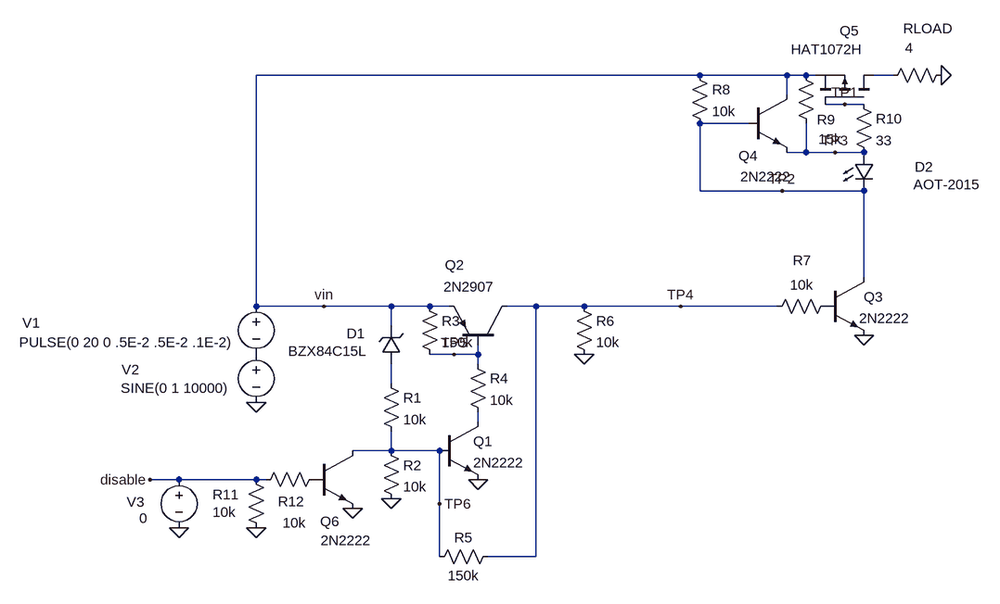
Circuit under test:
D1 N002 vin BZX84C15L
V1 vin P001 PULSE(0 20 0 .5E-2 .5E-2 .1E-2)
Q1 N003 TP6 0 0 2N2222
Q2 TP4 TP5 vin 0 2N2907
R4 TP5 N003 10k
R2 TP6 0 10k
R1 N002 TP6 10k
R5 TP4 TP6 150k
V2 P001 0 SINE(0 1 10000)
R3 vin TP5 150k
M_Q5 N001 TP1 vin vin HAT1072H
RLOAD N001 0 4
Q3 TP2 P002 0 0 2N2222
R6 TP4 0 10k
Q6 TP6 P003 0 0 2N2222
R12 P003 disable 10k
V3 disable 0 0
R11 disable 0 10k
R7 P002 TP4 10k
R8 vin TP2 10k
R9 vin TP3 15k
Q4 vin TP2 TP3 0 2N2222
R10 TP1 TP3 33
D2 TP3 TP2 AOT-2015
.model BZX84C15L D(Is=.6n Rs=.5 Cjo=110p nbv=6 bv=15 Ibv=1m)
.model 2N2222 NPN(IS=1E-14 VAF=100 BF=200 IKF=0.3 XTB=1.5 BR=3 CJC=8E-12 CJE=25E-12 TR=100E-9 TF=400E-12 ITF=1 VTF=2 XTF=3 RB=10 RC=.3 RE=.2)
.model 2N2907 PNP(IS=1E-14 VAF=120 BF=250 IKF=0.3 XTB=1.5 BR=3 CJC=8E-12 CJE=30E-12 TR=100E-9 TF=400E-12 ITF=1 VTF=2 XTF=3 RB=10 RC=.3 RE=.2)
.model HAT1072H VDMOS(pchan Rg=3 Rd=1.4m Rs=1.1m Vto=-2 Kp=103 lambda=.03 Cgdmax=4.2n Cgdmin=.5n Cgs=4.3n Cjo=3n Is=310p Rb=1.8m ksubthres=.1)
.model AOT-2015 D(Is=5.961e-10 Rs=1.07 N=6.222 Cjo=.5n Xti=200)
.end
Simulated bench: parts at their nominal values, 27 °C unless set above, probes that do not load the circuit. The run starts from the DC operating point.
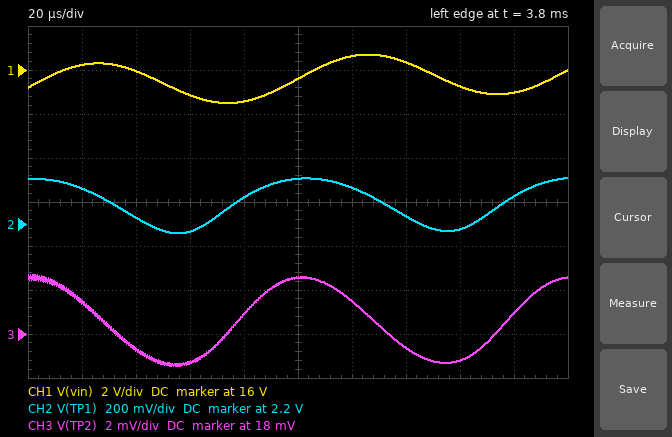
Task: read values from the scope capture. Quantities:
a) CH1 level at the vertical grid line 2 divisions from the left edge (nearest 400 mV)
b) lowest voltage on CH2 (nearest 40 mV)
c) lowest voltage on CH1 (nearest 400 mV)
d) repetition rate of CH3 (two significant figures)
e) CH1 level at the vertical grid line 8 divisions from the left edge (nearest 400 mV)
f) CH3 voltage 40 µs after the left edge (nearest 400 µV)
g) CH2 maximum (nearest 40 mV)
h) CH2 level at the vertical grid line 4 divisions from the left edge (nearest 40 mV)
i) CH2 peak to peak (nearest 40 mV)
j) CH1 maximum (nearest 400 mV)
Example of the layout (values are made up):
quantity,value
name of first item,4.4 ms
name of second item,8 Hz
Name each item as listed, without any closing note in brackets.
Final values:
quantity,value
CH1 level at the vertical grid line 2 divisions from the left edge,16.0 V
lowest voltage on CH2,2.16 V
lowest voltage on CH1,14.4 V
repetition rate of CH3,10 kHz
CH1 level at the vertical grid line 8 divisions from the left edge,15.2 V
CH3 voltage 40 µs after the left edge,17.2 mV
CH2 maximum,2.40 V
CH2 level at the vertical grid line 4 divisions from the left edge,2.32 V
CH2 peak to peak,240 mV
CH1 maximum,16.8 V
